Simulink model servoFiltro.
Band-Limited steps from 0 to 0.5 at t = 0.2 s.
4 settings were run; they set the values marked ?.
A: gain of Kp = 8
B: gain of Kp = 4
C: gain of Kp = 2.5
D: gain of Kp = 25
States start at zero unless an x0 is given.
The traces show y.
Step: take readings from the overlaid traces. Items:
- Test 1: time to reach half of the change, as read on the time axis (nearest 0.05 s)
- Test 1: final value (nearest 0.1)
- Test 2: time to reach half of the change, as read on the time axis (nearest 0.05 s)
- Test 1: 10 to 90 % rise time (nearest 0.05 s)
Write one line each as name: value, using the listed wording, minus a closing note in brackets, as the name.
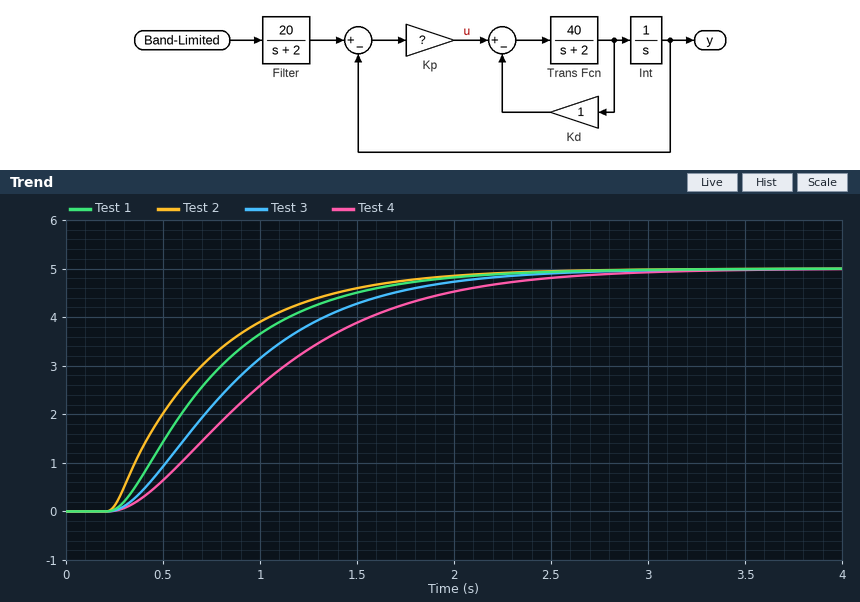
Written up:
Test 1: time to reach half of the change, as read on the time axis: 0.70 s
Test 1: final value: 5.0
Test 2: time to reach half of the change, as read on the time axis: 0.60 s
Test 1: 10 to 90 % rise time: 1.15 s
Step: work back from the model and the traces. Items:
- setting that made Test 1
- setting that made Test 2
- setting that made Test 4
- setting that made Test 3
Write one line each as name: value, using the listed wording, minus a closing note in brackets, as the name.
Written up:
setting that made Test 1: A
setting that made Test 2: D
setting that made Test 4: C
setting that made Test 3: B
